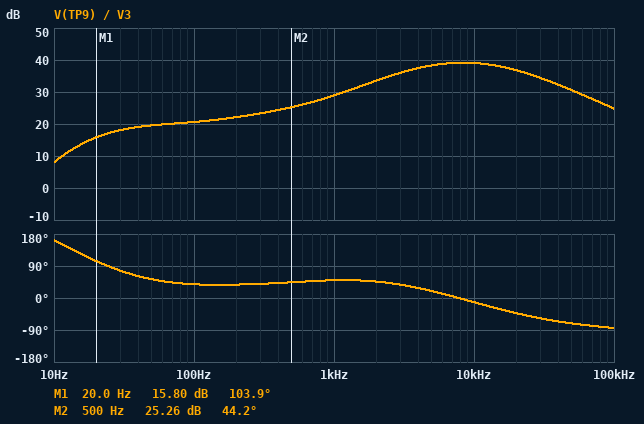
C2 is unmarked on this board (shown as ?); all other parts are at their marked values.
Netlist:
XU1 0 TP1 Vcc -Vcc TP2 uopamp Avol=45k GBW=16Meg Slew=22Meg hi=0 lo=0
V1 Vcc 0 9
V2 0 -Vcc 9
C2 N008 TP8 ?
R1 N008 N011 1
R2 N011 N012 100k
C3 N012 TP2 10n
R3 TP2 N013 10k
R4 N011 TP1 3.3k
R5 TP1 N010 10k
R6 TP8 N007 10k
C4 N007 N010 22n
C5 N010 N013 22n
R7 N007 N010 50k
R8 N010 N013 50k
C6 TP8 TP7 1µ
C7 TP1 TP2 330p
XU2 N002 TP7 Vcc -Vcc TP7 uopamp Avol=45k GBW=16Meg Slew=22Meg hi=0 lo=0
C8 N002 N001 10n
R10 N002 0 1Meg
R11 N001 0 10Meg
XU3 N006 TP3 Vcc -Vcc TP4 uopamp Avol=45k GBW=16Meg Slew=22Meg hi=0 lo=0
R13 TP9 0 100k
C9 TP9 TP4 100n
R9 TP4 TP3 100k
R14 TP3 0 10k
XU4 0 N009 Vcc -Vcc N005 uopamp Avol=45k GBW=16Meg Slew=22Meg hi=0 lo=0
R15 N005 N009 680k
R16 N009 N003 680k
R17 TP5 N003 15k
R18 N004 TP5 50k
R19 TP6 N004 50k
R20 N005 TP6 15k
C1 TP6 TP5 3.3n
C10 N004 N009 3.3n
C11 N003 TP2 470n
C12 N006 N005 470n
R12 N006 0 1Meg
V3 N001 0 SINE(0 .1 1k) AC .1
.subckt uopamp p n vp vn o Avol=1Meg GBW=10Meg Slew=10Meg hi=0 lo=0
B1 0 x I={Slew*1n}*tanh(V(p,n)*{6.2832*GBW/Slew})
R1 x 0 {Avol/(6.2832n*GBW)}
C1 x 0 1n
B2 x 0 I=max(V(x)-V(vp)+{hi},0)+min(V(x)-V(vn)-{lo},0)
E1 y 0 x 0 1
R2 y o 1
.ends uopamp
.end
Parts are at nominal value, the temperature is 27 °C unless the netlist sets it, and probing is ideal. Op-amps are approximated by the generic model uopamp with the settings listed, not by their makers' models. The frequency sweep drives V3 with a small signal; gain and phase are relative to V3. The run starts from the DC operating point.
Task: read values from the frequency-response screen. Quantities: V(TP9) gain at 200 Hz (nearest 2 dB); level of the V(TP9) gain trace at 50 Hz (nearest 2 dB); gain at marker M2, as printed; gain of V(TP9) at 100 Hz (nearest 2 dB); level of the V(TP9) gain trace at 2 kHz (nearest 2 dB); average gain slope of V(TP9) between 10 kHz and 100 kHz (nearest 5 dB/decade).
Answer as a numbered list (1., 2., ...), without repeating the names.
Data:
1. 22 dB
2. 20 dB
3. 25.26 dB
4. 20 dB
5. 34 dB
6. -15 dB/decade
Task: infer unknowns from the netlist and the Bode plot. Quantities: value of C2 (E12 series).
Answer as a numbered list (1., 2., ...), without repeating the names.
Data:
1. 15 nF
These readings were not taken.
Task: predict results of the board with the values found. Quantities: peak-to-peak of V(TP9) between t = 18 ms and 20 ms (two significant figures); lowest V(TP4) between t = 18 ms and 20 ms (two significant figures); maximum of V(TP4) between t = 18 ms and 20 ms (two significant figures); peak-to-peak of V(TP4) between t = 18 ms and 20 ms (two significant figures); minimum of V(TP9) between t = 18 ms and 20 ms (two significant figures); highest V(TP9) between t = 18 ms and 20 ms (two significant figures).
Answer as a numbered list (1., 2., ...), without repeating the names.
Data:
1. 5.6 V
2. -2.8 V
3. 2.8 V
4. 5.6 V
5. -2.8 V
6. 2.8 V
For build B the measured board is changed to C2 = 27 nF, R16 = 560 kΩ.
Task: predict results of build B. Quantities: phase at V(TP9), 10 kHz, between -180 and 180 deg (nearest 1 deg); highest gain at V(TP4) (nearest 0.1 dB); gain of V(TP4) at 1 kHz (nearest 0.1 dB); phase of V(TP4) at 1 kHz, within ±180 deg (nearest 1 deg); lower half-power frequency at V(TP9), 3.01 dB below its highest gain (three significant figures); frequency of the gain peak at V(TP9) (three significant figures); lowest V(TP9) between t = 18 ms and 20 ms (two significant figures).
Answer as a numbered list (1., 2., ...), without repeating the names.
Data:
1. -21 deg
2. 40.0 dB
3. 33.2 dB
4. 45 deg
5. 1.93 kHz
6. 6.29 kHz
7. -4.6 V
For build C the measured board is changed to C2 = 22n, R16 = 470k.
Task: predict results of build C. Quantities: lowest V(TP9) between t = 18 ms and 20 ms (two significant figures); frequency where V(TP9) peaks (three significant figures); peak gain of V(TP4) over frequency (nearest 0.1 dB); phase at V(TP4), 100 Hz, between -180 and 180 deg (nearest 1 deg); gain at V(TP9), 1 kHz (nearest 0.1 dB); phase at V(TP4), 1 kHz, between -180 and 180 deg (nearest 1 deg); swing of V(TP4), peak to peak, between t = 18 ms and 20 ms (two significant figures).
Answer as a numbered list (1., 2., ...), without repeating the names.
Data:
1. -4.0 V
2. 6.94 kHz
3. 40.0 dB
4. 28 deg
5. 32.0 dB
6. 45 deg
7. 8.0 V
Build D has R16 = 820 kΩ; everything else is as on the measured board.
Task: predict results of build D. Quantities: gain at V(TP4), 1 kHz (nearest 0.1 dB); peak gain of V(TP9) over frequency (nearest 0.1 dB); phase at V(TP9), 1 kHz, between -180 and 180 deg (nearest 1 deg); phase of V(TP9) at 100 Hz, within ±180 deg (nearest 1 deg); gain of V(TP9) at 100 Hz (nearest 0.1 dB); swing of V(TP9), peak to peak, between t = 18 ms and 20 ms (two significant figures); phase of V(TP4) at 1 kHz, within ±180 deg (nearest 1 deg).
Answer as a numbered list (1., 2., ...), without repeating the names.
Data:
1. 28.8 dB
2. 39.0 dB
3. 51 deg
4. 43 deg
5. 19.6 dB
6. 5.5 V
7. 50 deg
